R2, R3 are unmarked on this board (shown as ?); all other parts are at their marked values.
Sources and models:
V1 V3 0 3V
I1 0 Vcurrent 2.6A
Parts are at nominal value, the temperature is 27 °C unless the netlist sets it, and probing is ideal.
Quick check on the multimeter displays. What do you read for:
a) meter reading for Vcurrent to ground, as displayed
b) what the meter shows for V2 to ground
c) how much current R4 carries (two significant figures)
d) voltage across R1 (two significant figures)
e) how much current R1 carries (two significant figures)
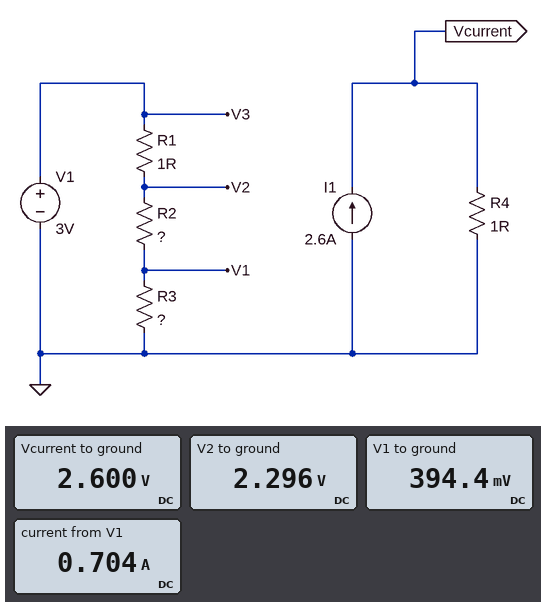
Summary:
2.600 V
2.296 V
2.6 A
700 mV
700 mA
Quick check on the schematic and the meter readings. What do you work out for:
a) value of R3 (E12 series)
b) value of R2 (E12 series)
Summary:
0.56 Ω
2.7 Ω
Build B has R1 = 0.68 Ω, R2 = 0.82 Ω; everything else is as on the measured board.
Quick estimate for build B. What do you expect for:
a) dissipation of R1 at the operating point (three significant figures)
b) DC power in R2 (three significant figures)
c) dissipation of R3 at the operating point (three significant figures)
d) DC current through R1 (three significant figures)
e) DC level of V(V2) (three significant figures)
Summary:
1.44 W
1.74 W
1.19 W
1.46 A
2.01 V
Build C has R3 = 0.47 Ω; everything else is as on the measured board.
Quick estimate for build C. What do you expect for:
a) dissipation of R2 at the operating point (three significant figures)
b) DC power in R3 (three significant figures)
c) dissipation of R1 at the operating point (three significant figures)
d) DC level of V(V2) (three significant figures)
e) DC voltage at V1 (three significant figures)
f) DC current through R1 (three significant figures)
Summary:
1.40 W
243 mW
518 mW
2.28 V
338 mV
719 mA
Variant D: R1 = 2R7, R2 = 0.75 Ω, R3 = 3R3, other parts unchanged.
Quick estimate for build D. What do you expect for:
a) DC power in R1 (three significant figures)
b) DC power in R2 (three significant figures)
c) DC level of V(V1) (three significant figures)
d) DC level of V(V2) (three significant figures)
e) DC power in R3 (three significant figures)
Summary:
533 mW
148 mW
1.47 V
1.80 V
652 mW
